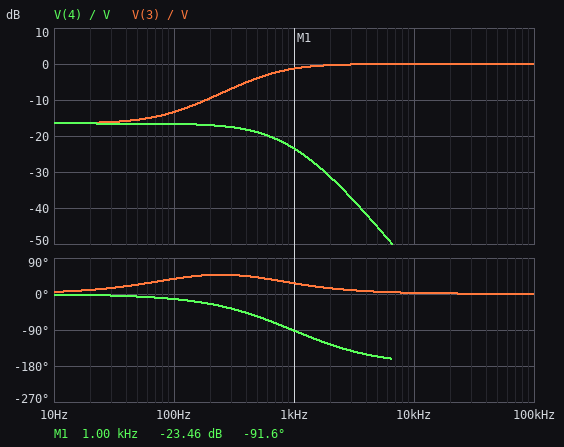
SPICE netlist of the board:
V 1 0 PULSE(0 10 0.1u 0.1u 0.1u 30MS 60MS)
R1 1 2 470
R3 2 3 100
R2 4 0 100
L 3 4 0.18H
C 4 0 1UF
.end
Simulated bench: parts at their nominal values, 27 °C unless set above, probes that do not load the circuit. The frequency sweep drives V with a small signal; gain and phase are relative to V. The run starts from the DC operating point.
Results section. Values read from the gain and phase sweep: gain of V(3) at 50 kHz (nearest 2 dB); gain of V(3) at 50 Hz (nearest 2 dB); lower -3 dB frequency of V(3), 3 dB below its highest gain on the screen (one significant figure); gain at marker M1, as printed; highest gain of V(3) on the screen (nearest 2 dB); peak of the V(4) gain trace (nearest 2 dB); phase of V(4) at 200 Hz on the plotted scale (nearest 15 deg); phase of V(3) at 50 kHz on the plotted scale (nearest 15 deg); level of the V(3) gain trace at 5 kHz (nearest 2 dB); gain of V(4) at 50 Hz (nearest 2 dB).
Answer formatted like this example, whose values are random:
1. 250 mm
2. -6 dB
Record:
1. 0 dB
2. -16 dB
3. 600 Hz
4. -23.46 dB
5. 0 dB
6. -16 dB
7. -30 deg
8. 0 deg
9. 0 dB
10. -16 dB
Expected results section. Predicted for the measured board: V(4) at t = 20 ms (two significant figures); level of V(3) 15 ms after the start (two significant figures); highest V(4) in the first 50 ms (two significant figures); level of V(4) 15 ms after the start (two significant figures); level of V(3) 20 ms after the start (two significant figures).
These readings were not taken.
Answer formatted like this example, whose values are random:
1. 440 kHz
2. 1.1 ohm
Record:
1. 1.5 V
2. 1.5 V
3. 1.5 V
4. 1.5 V
5. 1.5 V
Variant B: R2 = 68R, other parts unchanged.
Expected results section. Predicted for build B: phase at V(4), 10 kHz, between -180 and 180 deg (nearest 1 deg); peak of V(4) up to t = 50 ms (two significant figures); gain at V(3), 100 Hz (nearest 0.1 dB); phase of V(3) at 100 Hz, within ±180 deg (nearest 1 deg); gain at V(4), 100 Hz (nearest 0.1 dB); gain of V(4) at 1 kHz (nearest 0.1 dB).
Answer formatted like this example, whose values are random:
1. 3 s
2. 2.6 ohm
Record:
1. -164 deg
2. 1.1 V
3. -14.0 dB
4. 49 deg
5. -19.6 dB
6. -26.2 dB
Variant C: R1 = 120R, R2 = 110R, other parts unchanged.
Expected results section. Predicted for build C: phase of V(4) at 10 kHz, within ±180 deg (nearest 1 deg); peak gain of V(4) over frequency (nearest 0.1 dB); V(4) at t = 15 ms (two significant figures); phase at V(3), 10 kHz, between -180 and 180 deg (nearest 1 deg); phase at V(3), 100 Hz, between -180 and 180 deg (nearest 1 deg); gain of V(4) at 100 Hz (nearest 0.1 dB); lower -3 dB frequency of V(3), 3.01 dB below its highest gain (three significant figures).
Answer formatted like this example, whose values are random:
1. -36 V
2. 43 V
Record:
1. -171 deg
2. -9.5 dB
3. 3.3 V
4. 1 deg
5. 26 deg
6. -10.0 dB
7. 274 Hz
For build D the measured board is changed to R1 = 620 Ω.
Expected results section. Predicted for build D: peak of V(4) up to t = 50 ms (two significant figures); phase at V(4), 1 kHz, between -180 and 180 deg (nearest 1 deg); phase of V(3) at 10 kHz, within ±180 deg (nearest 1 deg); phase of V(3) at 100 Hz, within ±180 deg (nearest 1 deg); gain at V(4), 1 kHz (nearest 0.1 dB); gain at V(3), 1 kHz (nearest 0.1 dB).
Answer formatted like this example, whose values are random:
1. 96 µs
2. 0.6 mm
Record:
1. 1.2 V
2. -86 deg
3. 4 deg
4. 40 deg
5. -24.0 dB
6. -1.8 dB
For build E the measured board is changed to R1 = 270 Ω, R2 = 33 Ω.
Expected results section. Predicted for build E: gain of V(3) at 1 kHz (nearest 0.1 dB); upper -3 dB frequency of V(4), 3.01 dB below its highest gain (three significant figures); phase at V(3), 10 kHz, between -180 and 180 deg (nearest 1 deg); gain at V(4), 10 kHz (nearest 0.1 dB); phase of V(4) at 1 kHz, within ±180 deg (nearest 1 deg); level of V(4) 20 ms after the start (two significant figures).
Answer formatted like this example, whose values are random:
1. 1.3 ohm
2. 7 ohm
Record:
1. -0.5 dB
2. 357 Hz
3. 2 deg
4. -57.9 dB
5. -82 deg
6. 820 mV
